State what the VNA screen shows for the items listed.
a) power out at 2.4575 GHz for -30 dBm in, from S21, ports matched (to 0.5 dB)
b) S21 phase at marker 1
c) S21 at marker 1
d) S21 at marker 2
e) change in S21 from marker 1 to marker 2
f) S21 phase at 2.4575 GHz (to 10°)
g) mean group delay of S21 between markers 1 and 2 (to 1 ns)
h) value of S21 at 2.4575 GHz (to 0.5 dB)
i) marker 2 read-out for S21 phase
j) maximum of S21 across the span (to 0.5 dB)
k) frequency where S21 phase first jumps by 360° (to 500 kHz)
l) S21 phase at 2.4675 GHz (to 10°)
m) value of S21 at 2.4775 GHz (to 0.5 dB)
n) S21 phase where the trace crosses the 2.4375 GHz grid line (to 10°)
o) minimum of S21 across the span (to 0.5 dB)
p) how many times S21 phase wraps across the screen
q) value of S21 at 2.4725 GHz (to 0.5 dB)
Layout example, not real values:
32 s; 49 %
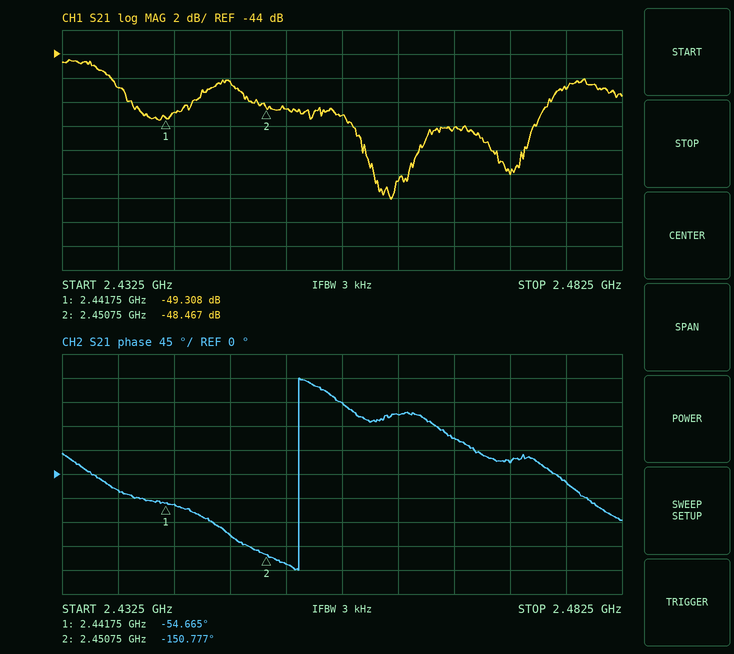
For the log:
-79.0 dBm; -54.665°; -49.308 dB; -48.467 dB; 0.841 dB; 130°; 30 ns; -49.0 dB; -150.777°; -44.5 dB; 2.4535 GHz; 70°; -47.0 dB; -30°; -56.0 dB; 1; -54.0 dB
